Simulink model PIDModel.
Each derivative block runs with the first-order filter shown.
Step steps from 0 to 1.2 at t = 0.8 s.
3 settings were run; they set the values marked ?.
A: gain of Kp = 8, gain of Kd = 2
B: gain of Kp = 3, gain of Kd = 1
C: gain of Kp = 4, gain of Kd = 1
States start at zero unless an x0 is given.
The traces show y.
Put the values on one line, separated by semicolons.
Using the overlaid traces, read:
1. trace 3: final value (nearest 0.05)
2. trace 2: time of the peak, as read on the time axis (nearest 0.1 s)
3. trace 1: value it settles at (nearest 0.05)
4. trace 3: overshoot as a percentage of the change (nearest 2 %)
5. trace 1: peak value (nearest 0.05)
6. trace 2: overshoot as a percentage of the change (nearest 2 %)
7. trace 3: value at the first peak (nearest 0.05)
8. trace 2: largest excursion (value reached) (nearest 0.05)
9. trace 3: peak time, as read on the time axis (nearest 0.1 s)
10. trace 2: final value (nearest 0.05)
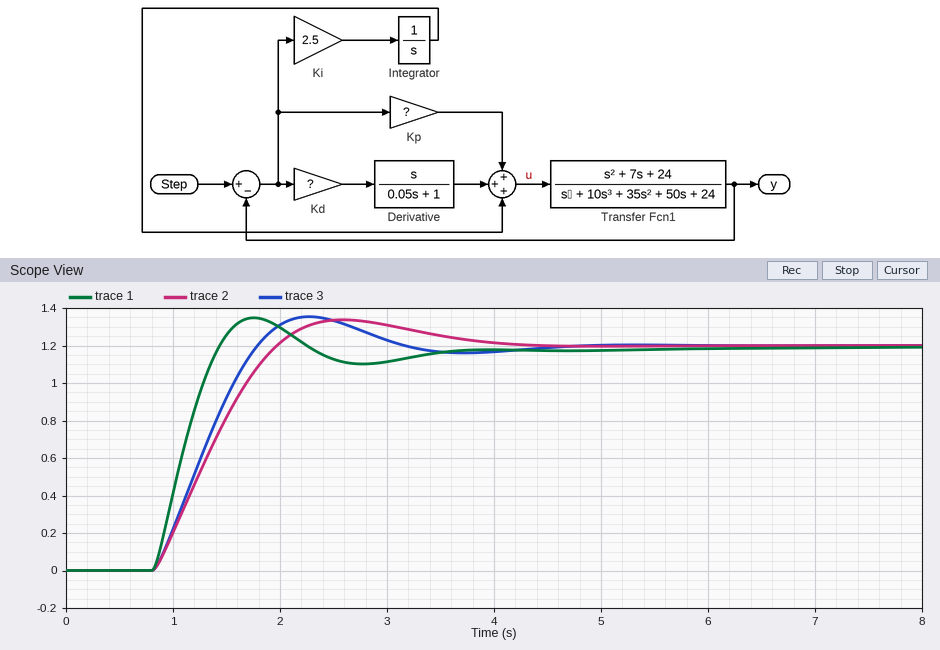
1.20; 2.6 s; 1.20; 12 %; 1.35; 12 %; 1.35; 1.35; 2.3 s; 1.20
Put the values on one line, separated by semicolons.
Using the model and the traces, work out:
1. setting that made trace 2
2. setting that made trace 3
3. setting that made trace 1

B; C; A
